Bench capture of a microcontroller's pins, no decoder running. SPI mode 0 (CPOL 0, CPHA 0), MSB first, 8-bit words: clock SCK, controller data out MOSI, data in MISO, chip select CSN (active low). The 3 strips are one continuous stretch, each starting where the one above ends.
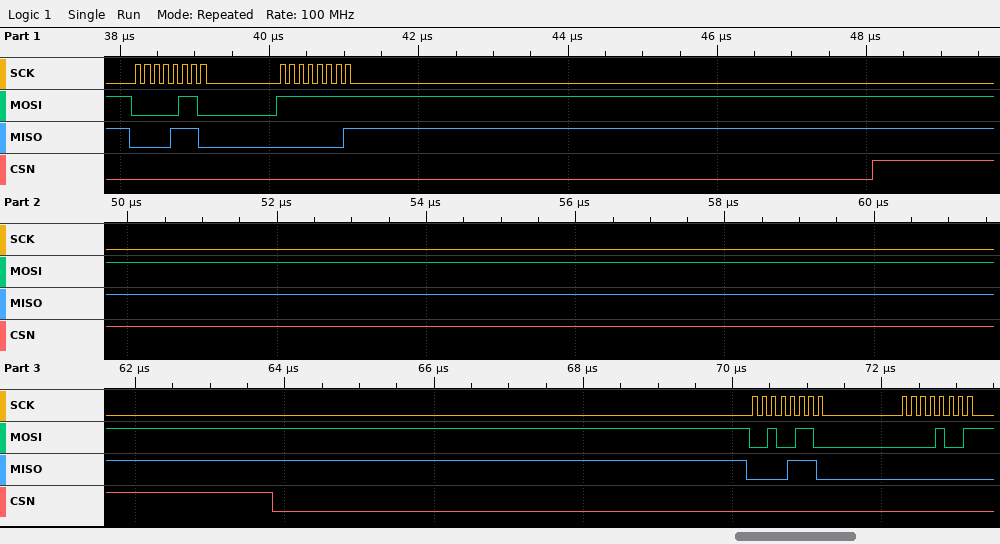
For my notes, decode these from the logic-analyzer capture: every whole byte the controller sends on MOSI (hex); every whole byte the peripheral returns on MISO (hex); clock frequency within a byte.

06 FF 26 09
0E 01 0E 00
8 MHz
